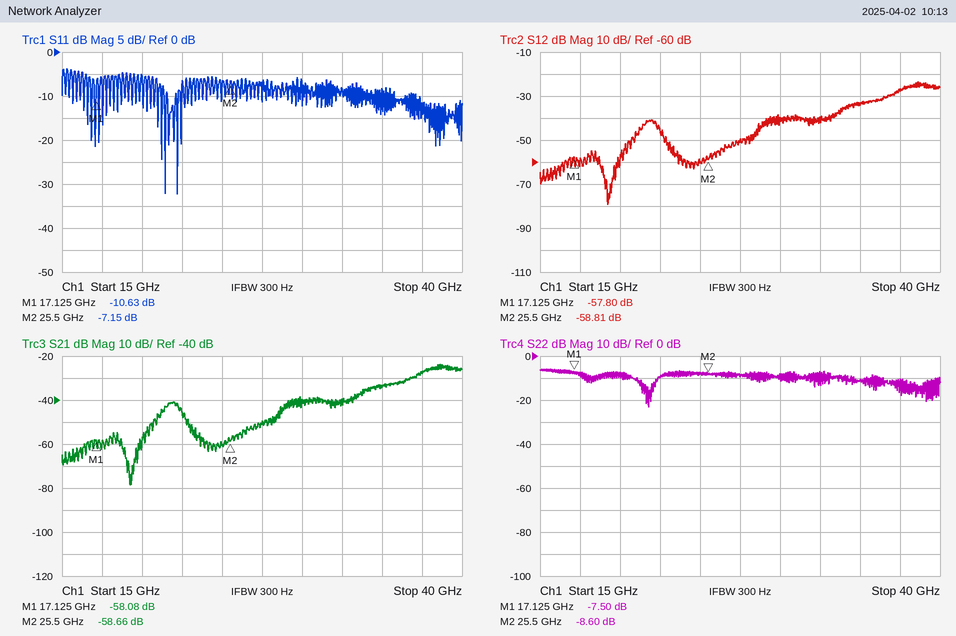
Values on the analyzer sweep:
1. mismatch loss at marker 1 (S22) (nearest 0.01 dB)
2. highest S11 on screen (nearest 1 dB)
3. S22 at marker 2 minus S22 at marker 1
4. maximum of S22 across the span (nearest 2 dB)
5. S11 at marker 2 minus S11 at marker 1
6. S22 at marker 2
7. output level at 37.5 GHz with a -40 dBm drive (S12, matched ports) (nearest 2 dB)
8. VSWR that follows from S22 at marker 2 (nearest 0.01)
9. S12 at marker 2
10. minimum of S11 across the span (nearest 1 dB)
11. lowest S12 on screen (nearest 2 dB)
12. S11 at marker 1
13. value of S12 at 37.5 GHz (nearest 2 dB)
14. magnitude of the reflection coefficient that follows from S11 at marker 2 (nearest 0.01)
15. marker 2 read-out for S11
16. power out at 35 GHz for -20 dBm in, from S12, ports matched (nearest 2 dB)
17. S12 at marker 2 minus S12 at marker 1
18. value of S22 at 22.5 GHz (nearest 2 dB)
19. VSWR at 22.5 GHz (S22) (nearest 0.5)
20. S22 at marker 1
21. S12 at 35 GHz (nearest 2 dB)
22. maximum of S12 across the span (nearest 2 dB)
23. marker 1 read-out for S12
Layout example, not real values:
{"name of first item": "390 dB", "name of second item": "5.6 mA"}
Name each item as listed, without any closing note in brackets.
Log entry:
{"mismatch loss at marker 1 (S22)": "0.85 dB", "highest S11 on screen": "-4 dB", "S22 at marker 2 minus S22 at marker 1": "-1.10 dB", "maximum of S22 across the span": "-6 dB", "S11 at marker 2 minus S11 at marker 1": "3.48 dB", "S22 at marker 2": "-8.60 dB", "output level at 37.5 GHz with a -40 dBm drive (S12, matched ports)": "-68 dBm", "VSWR that follows from S22 at marker 2": "2.18", "S12 at marker 2": "-58.81 dB", "minimum of S11 across the span": "-32 dB", "lowest S12 on screen": "-80 dB", "S11 at marker 1": "-10.63 dB", "value of S12 at 37.5 GHz": "-28 dB", "magnitude of the reflection coefficient that follows from S11 at marker 2": "0.44", "marker 2 read-out for S11": "-7.15 dB", "power out at 35 GHz for -20 dBm in, from S12, ports matched": "-54 dBm", "S12 at marker 2 minus S12 at marker 1": "-1.01 dB", "value of S22 at 22.5 GHz": "-10 dB", "VSWR at 22.5 GHz (S22)": "2.0", "S22 at marker 1": "-7.50 dB", "S12 at 35 GHz": "-34 dB", "maximum of S12 across the span": "-24 dB", "marker 1 read-out for S12": "-57.80 dB"}
